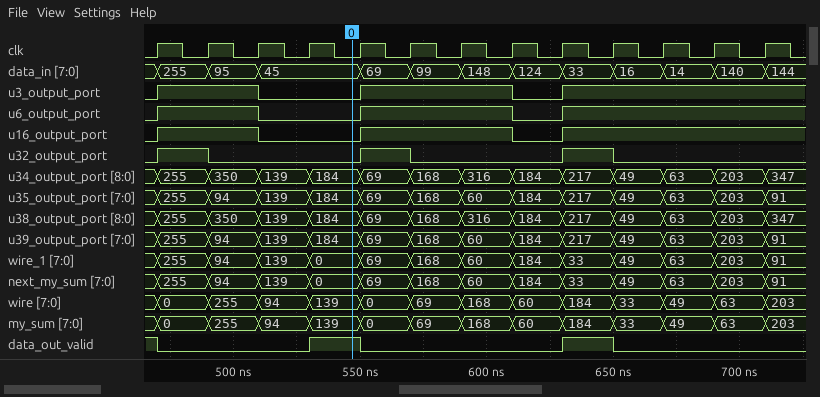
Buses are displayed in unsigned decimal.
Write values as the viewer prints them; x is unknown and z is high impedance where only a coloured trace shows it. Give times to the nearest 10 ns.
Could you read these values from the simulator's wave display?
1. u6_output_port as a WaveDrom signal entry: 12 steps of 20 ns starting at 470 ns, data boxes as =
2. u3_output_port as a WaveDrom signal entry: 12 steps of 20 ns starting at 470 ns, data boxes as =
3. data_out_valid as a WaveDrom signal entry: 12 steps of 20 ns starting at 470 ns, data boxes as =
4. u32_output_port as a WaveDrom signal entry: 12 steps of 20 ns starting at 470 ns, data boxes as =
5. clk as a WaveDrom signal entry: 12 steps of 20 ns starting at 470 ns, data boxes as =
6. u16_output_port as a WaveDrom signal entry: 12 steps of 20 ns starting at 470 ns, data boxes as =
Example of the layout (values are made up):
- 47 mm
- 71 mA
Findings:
- {name: 'u6_output_port', wave: '1.0.1..01...'}
- {name: 'u3_output_port', wave: '1.0.1..01...'}
- {name: 'data_out_valid', wave: '0..10...10..'}
- {name: 'u32_output_port', wave: '10..10..10..'}
- {name: 'clk', wave: 'p...........'}
- {name: 'u16_output_port', wave: '1.0.1..01...'}
